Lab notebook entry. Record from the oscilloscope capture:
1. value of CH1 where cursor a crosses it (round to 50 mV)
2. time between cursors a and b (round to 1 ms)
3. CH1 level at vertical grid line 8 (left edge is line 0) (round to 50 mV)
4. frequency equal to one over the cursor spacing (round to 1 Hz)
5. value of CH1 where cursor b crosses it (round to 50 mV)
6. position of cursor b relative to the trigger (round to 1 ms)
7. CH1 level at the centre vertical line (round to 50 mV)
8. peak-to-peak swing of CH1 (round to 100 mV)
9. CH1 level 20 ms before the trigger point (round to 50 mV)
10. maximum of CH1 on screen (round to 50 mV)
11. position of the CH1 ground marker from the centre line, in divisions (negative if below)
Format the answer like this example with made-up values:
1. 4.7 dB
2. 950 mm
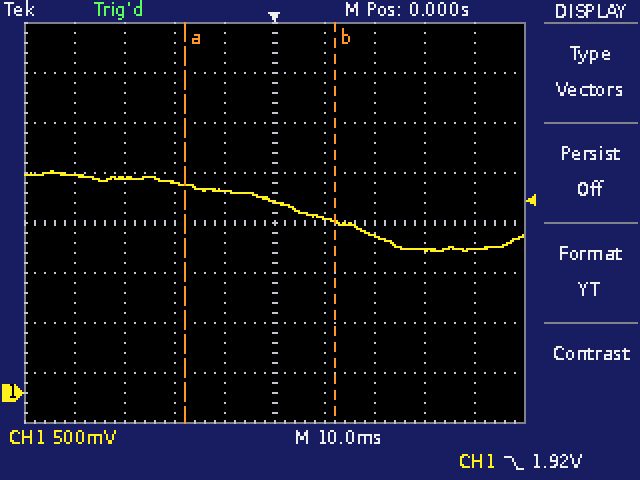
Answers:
1. 2.10 V
2. 30 ms
3. 1.45 V
4. 33 Hz
5. 1.70 V
6. +12 ms
7. 1.90 V
8. 800 mV
9. 2.10 V
10. 2.20 V
11. -3.4 div
